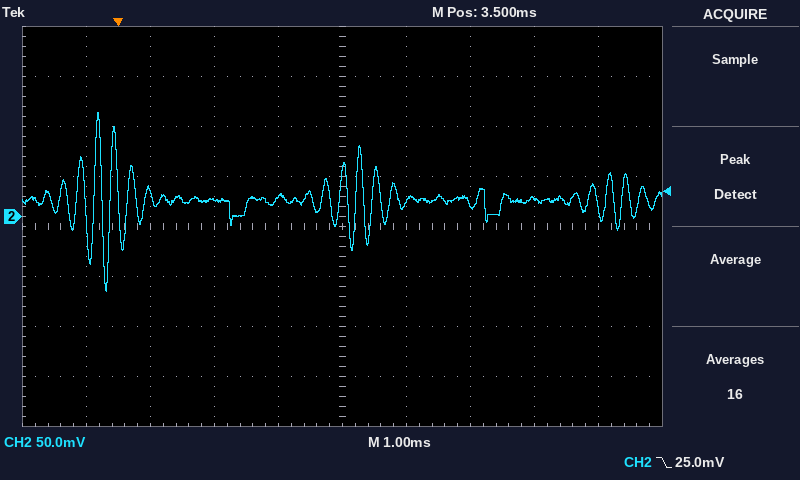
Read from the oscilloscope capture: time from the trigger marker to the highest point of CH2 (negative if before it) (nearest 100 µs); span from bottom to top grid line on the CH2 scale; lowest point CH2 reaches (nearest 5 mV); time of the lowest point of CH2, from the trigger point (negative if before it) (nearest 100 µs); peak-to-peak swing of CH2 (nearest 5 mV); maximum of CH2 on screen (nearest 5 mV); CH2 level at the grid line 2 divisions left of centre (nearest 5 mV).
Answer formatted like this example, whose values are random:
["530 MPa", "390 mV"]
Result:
["-300 µs", "400 mV", "-75 mV", "-200 µs", "180 mV", "105 mV", "15 mV"]
